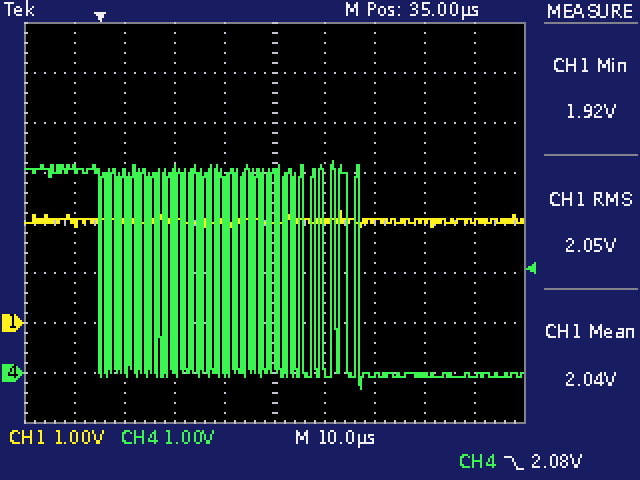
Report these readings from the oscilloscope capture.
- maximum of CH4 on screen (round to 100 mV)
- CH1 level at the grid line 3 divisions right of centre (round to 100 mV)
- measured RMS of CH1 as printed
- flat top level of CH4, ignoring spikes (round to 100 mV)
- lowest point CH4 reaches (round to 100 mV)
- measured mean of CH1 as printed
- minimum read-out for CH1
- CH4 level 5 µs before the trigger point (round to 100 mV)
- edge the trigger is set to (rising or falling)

4.2 V
2.0 V
2.05 V
4.1 V
-300 mV
2.04 V
1.92 V
4.1 V
falling
